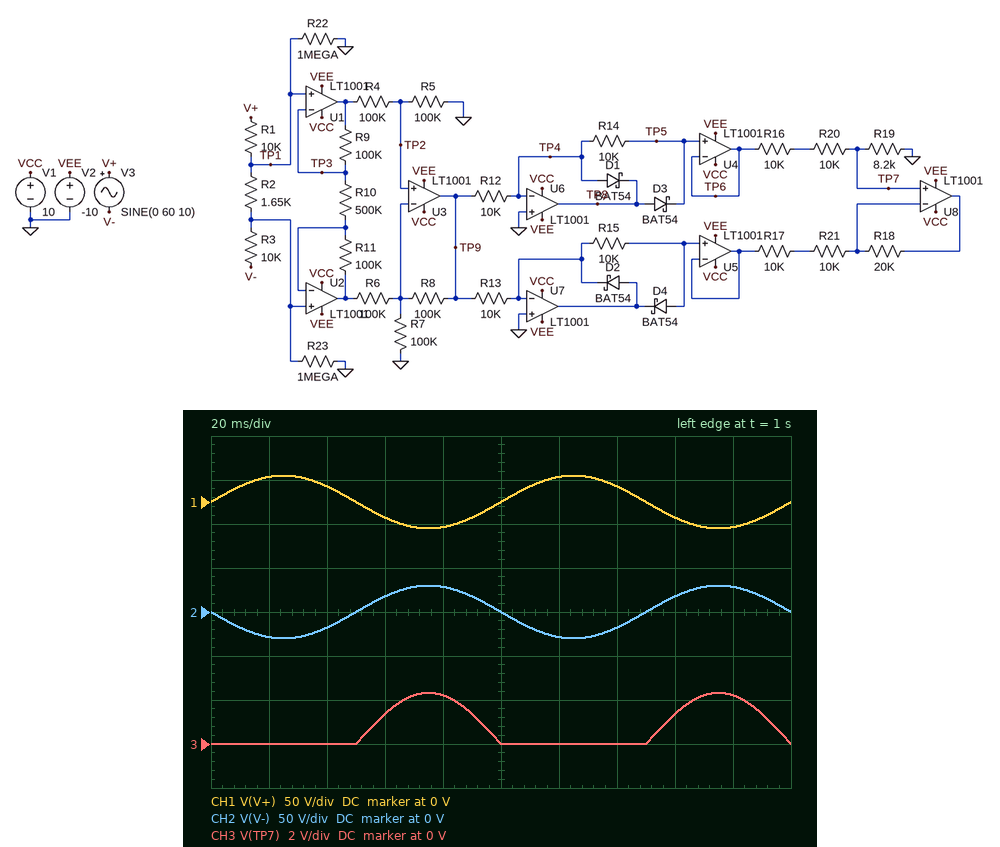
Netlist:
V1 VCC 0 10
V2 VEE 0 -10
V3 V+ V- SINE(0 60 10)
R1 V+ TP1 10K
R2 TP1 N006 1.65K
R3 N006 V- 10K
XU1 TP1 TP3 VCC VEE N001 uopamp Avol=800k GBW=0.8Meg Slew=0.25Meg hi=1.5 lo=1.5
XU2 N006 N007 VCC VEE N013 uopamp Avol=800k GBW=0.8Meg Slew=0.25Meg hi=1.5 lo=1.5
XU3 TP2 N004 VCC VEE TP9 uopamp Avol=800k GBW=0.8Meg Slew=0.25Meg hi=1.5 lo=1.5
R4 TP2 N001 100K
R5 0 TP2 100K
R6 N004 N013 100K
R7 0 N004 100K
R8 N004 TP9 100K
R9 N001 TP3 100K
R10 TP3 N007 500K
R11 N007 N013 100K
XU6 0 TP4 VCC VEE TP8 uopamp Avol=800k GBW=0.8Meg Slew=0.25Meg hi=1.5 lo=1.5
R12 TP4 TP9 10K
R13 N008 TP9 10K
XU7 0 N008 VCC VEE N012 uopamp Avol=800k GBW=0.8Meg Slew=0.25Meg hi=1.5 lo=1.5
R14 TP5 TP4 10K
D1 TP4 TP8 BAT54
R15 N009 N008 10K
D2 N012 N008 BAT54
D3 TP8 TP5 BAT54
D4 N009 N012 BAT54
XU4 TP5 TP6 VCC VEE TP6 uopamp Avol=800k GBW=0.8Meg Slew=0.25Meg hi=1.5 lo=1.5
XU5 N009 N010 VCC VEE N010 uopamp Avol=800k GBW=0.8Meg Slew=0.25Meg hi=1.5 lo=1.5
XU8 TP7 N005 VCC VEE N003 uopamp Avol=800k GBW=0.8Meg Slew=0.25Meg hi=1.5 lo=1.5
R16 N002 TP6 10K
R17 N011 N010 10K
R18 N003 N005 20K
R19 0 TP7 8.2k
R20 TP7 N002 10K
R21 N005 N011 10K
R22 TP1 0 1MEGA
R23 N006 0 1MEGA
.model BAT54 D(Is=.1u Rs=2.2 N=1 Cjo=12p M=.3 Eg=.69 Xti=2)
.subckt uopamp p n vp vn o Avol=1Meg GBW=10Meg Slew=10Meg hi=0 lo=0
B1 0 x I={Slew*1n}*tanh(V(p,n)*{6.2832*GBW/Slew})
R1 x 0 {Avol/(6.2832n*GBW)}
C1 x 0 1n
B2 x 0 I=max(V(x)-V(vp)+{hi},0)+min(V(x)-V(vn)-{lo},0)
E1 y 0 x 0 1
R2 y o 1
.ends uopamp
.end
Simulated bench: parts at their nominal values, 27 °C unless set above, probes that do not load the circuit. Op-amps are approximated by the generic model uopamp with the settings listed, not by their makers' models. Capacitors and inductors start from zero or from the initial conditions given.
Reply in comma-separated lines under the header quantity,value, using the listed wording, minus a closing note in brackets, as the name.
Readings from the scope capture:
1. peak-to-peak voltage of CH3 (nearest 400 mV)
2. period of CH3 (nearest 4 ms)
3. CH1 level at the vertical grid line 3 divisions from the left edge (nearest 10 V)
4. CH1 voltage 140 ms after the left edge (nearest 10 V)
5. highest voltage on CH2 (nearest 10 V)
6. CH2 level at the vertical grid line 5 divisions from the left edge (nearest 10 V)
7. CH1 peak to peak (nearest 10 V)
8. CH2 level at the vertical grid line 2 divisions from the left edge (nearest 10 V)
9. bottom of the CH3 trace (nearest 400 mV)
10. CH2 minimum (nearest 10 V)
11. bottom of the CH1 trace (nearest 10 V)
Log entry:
quantity,value
peak-to-peak voltage of CH3,2.4 V
period of CH3,100 ms
CH1 level at the vertical grid line 3 divisions from the left edge,-20 V
CH1 voltage 140 ms after the left edge,20 V
highest voltage on CH2,30 V
CH2 level at the vertical grid line 5 divisions from the left edge,0 V
CH1 peak to peak,60 V
CH2 level at the vertical grid line 2 divisions from the left edge,-20 V
bottom of the CH3 trace,0 V
CH2 minimum,-30 V
bottom of the CH1 trace,-30 V
